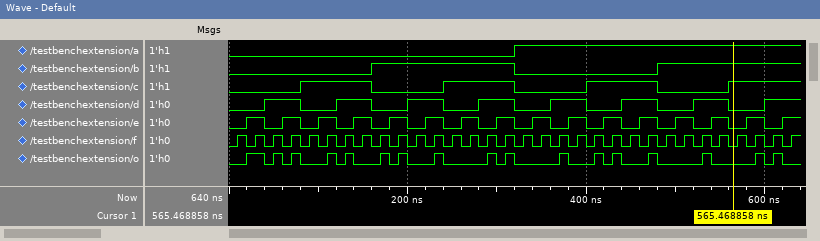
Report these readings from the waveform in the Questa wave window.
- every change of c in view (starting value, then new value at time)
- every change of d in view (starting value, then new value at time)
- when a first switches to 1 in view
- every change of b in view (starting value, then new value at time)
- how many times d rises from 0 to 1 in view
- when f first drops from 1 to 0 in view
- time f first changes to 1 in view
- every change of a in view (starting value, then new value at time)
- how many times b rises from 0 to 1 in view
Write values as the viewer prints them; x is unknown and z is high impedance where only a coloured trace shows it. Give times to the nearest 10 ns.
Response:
0, 1 at 80 ns, 0 at 160 ns, 1 at 240 ns, 0 at 320 ns, 1 at 400 ns, 0 at 480 ns, 1 at 560 ns
0, 1 at 40 ns, 0 at 80 ns, 1 at 120 ns, 0 at 160 ns, 1 at 200 ns, 0 at 240 ns, 1 at 280 ns, 0 at 320 ns, 1 at 360 ns, 0 at 400 ns, 1 at 440 ns, 0 at 480 ns, 1 at 520 ns, 0 at 560 ns, 1 at 600 ns
320 ns
0, 1 at 160 ns, 0 at 320 ns, 1 at 480 ns
8
20 ns
10 ns
0, 1 at 320 ns
2
